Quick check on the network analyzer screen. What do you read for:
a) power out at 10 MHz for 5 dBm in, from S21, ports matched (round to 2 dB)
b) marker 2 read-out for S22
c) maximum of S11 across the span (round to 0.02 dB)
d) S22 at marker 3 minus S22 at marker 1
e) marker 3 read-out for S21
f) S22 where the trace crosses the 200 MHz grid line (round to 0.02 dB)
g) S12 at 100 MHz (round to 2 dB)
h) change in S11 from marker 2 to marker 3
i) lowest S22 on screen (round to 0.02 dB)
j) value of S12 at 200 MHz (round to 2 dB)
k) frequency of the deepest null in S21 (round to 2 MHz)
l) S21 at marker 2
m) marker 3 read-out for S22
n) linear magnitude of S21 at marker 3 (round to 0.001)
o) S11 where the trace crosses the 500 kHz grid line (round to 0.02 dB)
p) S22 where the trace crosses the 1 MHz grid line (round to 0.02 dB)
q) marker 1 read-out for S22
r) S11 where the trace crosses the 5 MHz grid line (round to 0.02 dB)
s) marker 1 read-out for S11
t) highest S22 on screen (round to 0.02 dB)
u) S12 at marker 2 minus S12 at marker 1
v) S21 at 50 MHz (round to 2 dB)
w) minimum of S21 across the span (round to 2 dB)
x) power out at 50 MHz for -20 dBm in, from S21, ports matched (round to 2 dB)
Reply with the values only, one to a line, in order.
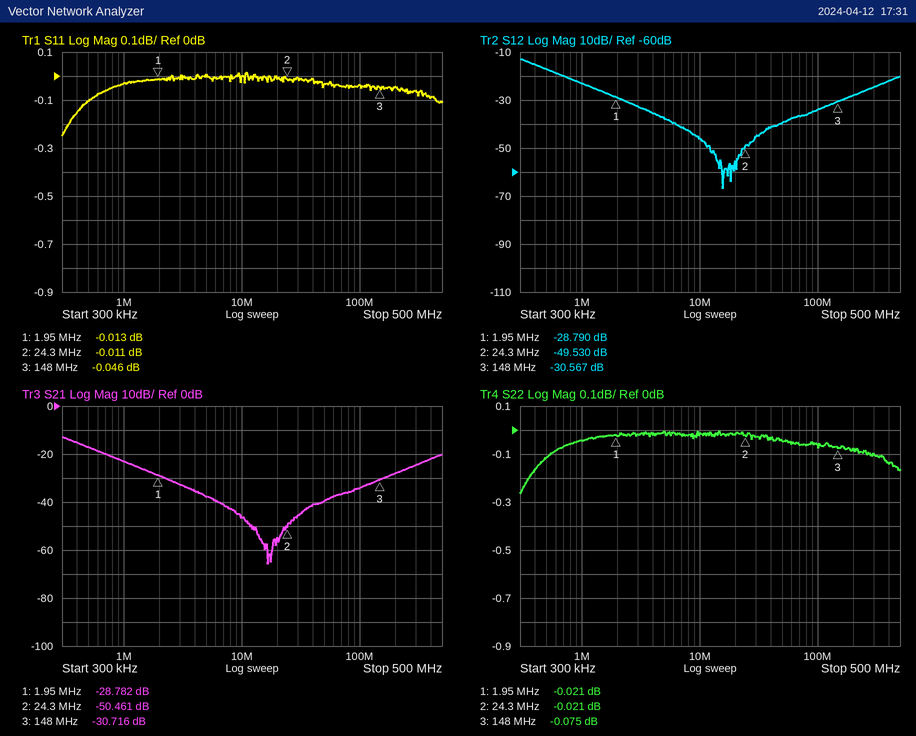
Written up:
-42 dBm
-0.021 dB
0.02 dB
-0.054 dB
-30.716 dB
-0.08 dB
-34 dB
-0.035 dB
-0.26 dB
-28 dB
16 MHz
-50.461 dB
-0.075 dB
0.029
-0.10 dB
-0.04 dB
-0.021 dB
0.00 dB
-0.013 dB
0.00 dB
-20.740 dB
-40 dB
-66 dB
-60 dBm
